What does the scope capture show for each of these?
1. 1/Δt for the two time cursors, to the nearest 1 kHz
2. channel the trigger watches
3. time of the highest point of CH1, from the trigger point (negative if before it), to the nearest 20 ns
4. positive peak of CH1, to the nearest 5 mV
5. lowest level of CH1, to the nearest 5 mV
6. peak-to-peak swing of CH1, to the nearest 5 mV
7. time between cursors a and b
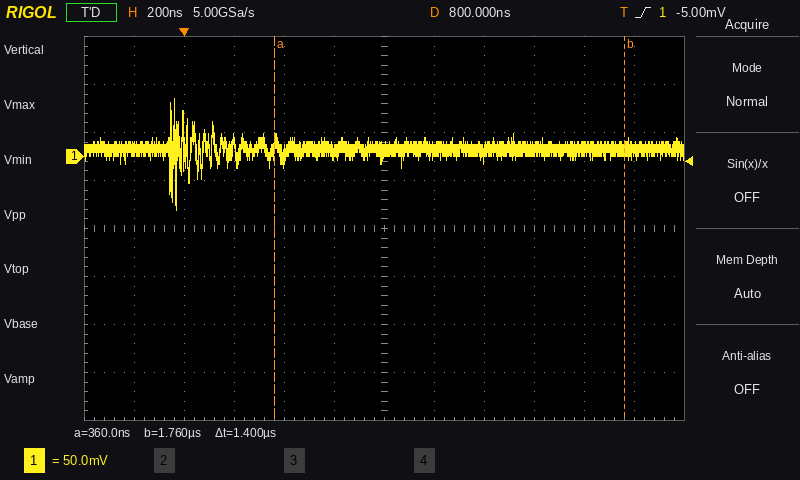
714 kHz
CH1
-40 ns
60 mV
-55 mV
115 mV
1.4 µs
